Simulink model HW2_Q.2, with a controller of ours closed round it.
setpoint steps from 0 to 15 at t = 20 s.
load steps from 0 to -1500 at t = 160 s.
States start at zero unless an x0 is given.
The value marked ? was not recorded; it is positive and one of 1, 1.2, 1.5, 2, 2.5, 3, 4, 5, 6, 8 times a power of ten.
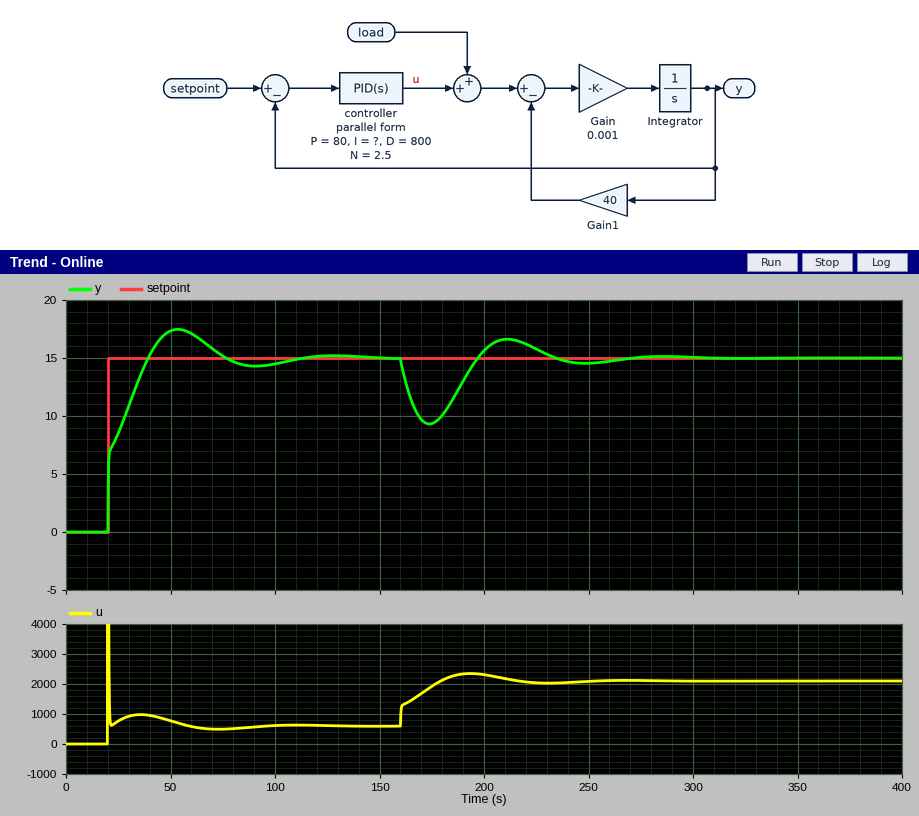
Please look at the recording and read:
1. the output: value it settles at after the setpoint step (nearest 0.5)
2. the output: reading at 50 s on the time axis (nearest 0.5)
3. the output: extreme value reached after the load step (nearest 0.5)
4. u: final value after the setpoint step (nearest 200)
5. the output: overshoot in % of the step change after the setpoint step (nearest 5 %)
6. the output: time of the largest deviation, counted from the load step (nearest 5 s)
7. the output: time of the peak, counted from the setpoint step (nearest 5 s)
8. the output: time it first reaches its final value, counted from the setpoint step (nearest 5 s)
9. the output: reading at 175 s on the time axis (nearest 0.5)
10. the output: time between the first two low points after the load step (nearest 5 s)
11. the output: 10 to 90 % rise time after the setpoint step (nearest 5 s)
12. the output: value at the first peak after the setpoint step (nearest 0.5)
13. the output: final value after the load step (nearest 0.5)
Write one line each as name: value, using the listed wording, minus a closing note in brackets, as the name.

the output: value it settles at after the setpoint step: 15.0
the output: reading at 50 s on the time axis: 17.5
the output: extreme value reached after the load step: 9.5
u: final value after the setpoint step: 600
the output: overshoot in % of the step change after the setpoint step: 15 %
the output: time of the largest deviation, counted from the load step: 15 s
the output: time of the peak, counted from the setpoint step: 35 s
the output: time it first reaches its final value, counted from the setpoint step: 20 s
the output: reading at 175 s on the time axis: 9.5
the output: time between the first two low points after the load step: 75 s
the output: 10 to 90 % rise time after the setpoint step: 15 s
the output: value at the first peak after the setpoint step: 17.5
the output: final value after the load step: 15.0
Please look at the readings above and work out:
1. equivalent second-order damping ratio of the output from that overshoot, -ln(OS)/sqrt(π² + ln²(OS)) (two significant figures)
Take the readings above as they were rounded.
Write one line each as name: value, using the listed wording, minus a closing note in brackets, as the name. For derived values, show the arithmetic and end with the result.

equivalent second-order damping ratio of the output from that overshoot, -ln(OS)/sqrt(π² + ln²(OS)): ln(0.15) = -1.897; 1.897 / sqrt(9.870 + 3.599) = 0.52
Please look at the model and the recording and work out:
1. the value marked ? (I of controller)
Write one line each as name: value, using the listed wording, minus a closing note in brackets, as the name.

the value marked ?: 15
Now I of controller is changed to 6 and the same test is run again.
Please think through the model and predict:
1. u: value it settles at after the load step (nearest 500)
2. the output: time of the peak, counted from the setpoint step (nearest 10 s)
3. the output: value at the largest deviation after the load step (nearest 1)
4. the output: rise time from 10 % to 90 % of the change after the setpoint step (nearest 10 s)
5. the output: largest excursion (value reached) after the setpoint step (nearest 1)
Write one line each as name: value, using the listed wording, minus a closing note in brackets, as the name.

u: value it settles at after the load step: 2000
the output: time of the peak, counted from the setpoint step: 60 s
the output: value at the largest deviation after the load step: 8
the output: rise time from 10 % to 90 % of the change after the setpoint step: 30 s
the output: largest excursion (value reached) after the setpoint step: 16
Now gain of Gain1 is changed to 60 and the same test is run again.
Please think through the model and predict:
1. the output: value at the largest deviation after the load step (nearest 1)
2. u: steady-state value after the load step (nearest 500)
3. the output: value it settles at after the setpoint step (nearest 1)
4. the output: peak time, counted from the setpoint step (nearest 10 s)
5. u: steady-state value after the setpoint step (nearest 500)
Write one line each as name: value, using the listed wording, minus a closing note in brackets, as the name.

the output: value at the largest deviation after the load step: 10
u: steady-state value after the load step: 2500
the output: value it settles at after the setpoint step: 15
the output: peak time, counted from the setpoint step: 40 s
u: steady-state value after the setpoint step: 1000
